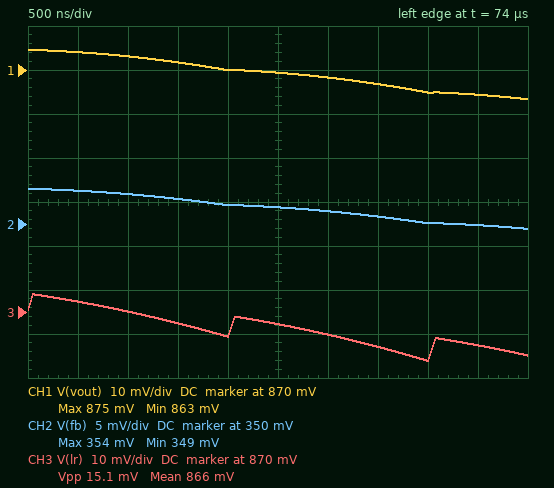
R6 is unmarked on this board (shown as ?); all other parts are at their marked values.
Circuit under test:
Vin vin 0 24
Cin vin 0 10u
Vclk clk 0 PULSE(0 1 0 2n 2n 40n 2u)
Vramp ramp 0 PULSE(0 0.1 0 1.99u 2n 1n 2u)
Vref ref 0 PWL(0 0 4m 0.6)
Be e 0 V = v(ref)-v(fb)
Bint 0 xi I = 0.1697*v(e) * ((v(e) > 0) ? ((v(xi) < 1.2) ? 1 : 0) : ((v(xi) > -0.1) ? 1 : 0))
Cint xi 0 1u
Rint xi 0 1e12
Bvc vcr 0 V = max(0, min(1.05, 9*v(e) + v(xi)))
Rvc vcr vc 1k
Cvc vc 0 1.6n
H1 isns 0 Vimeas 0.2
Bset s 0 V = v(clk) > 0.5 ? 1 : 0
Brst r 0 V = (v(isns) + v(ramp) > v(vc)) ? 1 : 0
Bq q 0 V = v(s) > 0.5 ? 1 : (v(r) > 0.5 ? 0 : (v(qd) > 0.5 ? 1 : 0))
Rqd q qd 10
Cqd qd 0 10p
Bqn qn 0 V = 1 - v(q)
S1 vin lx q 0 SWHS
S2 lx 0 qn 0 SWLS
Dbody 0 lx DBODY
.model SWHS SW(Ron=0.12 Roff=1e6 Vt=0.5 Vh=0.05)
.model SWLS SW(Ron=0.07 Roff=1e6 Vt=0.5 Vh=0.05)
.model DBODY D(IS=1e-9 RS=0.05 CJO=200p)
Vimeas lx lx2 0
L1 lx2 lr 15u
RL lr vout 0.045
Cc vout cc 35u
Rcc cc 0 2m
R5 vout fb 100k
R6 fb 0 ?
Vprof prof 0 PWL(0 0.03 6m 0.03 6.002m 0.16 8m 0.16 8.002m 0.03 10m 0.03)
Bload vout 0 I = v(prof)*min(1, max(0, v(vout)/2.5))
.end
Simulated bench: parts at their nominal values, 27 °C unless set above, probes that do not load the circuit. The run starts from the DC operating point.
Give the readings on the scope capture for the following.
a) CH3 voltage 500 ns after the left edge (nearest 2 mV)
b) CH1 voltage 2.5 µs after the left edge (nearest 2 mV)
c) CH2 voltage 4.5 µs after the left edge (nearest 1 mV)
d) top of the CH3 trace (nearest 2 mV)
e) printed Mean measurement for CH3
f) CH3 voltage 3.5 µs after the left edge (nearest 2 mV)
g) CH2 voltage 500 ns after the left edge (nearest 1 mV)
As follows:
872 mV
870 mV
350 mV
874 mV
866 mV
862 mV
354 mV
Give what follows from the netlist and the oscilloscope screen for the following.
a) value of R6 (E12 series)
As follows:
68 kΩ
